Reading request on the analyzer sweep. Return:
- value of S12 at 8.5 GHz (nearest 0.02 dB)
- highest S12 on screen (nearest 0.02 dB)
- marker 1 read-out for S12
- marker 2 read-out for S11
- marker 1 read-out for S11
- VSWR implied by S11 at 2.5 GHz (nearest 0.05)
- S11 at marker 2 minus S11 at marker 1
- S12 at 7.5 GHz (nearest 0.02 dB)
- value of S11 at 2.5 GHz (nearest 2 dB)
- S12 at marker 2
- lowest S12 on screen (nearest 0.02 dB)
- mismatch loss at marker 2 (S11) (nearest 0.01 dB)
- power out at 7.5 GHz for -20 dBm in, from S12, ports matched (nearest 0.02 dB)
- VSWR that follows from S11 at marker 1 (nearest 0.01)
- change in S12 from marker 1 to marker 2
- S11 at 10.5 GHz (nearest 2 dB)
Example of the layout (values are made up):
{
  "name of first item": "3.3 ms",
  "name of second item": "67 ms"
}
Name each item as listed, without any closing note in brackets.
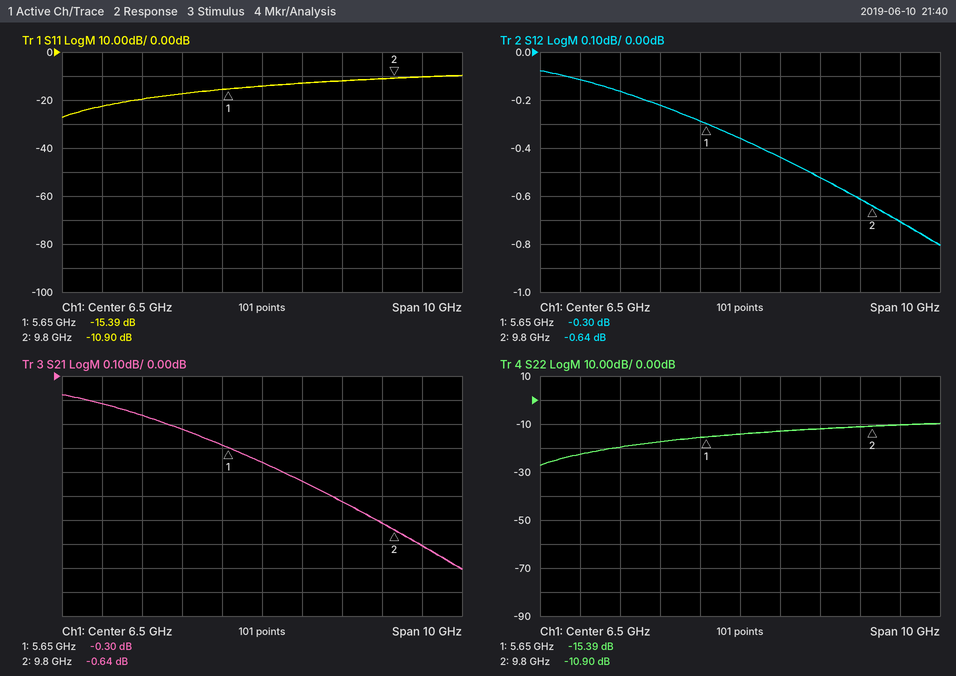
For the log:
{
  "value of S12 at 8.5 GHz": "-0.52 dB",
  "highest S12 on screen": "-0.08 dB",
  "marker 1 read-out for S12": "-0.30 dB",
  "marker 2 read-out for S11": "-10.90 dB",
  "marker 1 read-out for S11": "-15.39 dB",
  "VSWR implied by S11 at 2.5 GHz": "1.15",
  "S11 at marker 2 minus S11 at marker 1": "4.49 dB",
  "S12 at 7.5 GHz": "-0.44 dB",
  "value of S11 at 2.5 GHz": "-22 dB",
  "S12 at marker 2": "-0.64 dB",
  "lowest S12 on screen": "-0.80 dB",
  "mismatch loss at marker 2 (S11)": "0.37 dB",
  "power out at 7.5 GHz for -20 dBm in, from S12, ports matched": "-20.44 dBm",
  "VSWR that follows from S11 at marker 1": "1.41",
  "change in S12 from marker 1 to marker 2": "-0.34 dB",
  "S11 at 10.5 GHz": "-10 dB"
}
